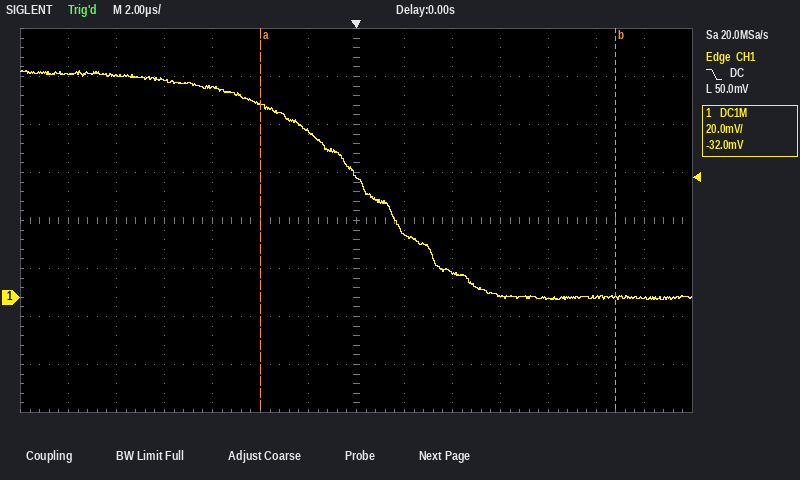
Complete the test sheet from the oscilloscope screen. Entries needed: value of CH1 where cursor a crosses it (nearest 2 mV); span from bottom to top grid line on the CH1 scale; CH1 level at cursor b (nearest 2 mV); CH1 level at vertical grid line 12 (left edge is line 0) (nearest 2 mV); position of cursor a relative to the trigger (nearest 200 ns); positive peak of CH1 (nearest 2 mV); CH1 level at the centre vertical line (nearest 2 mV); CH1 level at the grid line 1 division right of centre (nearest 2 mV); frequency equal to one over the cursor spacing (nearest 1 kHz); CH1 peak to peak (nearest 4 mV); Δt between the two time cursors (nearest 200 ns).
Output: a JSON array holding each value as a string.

["80 mV", "160 mV", "0 mV", "0 mV", "-4.0 µs", "94 mV", "50 mV", "26 mV", "68 kHz", "96 mV", "14.8 µs"]
